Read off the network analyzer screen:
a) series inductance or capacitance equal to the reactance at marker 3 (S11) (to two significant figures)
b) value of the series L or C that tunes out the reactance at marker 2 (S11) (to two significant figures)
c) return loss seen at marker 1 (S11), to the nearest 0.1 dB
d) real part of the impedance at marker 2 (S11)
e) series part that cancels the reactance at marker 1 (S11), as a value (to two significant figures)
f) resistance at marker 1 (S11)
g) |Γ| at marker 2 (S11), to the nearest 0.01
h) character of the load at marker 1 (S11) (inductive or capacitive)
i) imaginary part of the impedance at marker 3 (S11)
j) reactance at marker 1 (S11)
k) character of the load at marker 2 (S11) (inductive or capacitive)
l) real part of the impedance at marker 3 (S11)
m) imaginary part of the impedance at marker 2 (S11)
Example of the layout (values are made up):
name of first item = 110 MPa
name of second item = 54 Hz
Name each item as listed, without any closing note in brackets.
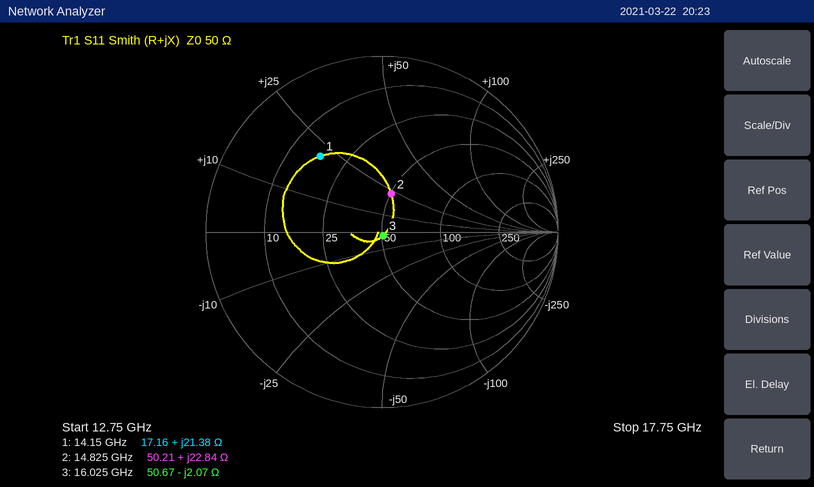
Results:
series inductance or capacitance equal to the reactance at marker 3 (S11) = 4.8 pF
value of the series L or C that tunes out the reactance at marker 2 (S11) = 470 fF
return loss seen at marker 1 (S11), to the nearest 0.1 dB = 5.1 dB
real part of the impedance at marker 2 = 50.21 Ω
series part that cancels the reactance at marker 1 (S11), as a value = 530 fF
resistance at marker 1 = 17.16 Ω
|Γ| at marker 2 (S11), to the nearest 0.01 = 0.22
character of the load at marker 1 (S11) = inductive
imaginary part of the impedance at marker 3 = -2.07 Ω
reactance at marker 1 = +21.38 Ω
character of the load at marker 2 (S11) = inductive
real part of the impedance at marker 3 = 50.67 Ω
imaginary part of the impedance at marker 2 = +22.84 Ω
